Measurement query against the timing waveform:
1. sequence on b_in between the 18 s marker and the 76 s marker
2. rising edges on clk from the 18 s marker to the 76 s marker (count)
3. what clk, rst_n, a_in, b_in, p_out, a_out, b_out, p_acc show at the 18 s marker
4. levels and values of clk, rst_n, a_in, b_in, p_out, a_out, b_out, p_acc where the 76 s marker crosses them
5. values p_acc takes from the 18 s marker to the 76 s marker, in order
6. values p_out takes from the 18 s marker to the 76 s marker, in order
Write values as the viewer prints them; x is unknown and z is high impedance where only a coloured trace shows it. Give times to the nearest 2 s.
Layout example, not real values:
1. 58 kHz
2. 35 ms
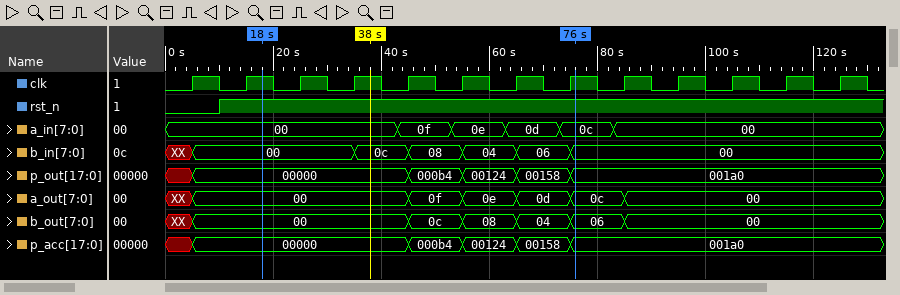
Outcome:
1. 00, 0c, 08, 04, 06, 00
2. 6
3. clk=1, rst_n=1, a_in=00, b_in=00, p_out=00000, a_out=00, b_out=00, p_acc=00000
4. clk=1, rst_n=1, a_in=0c, b_in=00, p_out=001a0, a_out=0c, b_out=06, p_acc=001a0
5. 00000, 000b4, 00124, 00158, 001a0
6. 00000, 000b4, 00124, 00158, 001a0
